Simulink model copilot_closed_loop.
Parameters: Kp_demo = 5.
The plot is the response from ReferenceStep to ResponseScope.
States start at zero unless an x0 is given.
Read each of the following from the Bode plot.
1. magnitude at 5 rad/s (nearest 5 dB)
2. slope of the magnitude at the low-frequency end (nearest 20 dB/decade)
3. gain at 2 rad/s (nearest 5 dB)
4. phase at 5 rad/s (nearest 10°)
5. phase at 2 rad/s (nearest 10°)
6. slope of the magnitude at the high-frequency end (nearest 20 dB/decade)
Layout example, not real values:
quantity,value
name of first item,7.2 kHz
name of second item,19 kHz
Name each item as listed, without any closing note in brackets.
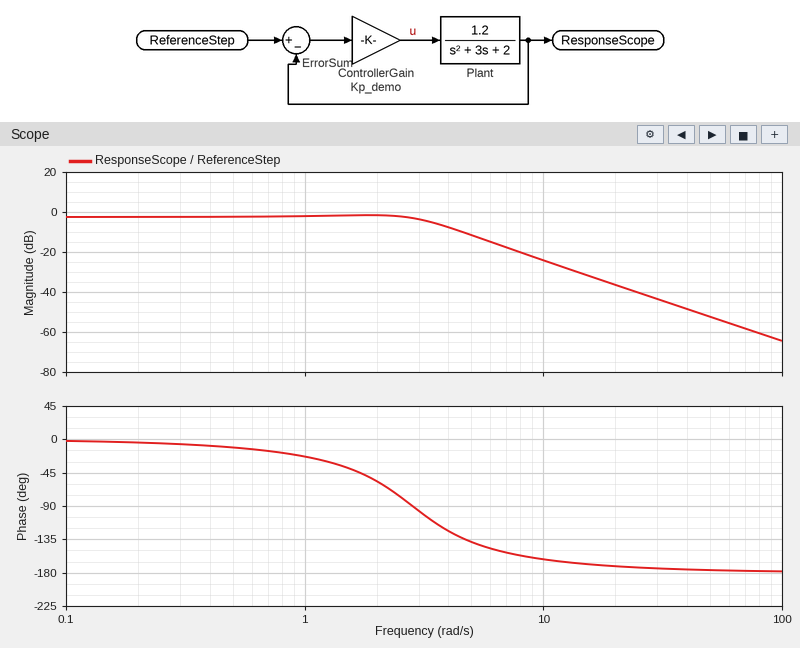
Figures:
quantity,value
magnitude at 5 rad/s,-10 dB
slope of the magnitude at the low-frequency end,0 dB/decade
gain at 2 rad/s,0 dB
phase at 5 rad/s,-140°
phase at 2 rad/s,-60°
slope of the magnitude at the high-frequency end,-40 dB/decade
